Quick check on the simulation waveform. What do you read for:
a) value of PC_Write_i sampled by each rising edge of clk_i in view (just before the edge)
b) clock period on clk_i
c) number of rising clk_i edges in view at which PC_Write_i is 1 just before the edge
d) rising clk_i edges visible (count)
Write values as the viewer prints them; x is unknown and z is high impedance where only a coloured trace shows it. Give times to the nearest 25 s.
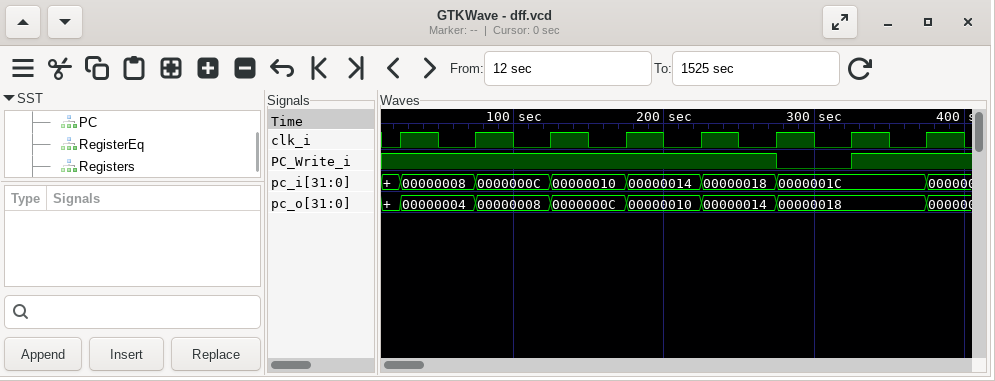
1 1 1 1 1 1 0 1
50 s
7
8
